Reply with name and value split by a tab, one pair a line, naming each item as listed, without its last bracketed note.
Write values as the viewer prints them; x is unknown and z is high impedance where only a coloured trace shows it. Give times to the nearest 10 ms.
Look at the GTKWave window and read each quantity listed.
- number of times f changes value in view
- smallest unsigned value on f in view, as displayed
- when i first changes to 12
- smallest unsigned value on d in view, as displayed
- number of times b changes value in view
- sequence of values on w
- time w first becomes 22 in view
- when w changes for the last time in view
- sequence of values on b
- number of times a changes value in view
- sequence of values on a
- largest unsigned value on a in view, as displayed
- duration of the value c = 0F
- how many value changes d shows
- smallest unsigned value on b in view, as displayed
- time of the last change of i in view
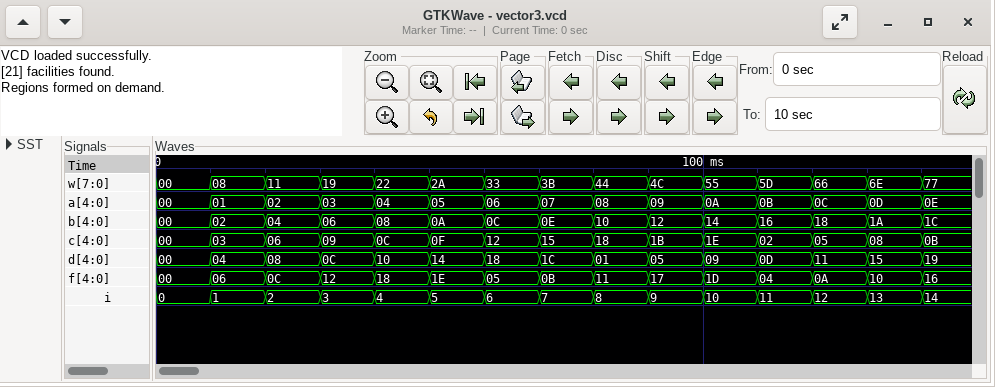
number of times f changes value in view	14
smallest unsigned value on f in view, as displayed	00
when i first changes to 12	120 ms
smallest unsigned value on d in view, as displayed	00
number of times b changes value in view	14
sequence of values on w	00, 08, 11, 19, 22, 2A, 33, 3B, 44, 4C, 55, 5D, 66, 6E, 77
time w first becomes 22 in view	40 ms
when w changes for the last time in view	140 ms
sequence of values on b	00, 02, 04, 06, 08, 0A, 0C, 0E, 10, 12, 14, 16, 18, 1A, 1C
number of times a changes value in view	14
sequence of values on a	00, 01, 02, 03, 04, 05, 06, 07, 08, 09, 0A, 0B, 0C, 0D, 0E
largest unsigned value on a in view, as displayed	0E
duration of the value c = 0F	10 ms
how many value changes d shows	14
smallest unsigned value on b in view, as displayed	00
time of the last change of i in view	140 ms
